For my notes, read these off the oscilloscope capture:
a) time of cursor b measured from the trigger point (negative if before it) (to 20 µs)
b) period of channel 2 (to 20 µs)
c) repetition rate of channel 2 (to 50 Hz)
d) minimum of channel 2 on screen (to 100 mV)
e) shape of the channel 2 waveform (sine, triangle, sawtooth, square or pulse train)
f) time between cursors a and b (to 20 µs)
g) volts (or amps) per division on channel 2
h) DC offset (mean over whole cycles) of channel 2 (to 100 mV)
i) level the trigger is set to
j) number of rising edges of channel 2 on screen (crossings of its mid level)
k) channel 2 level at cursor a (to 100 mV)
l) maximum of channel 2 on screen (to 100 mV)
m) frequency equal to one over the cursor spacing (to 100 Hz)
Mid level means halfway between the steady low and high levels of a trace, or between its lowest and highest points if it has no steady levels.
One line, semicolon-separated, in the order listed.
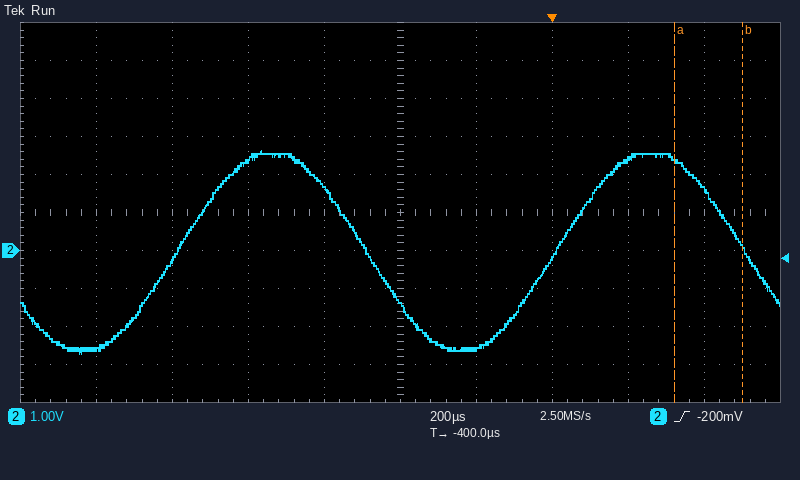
+500 µs; 1.00 ms; 1.00 kHz; -2.7 V; sine; 180 µs; 1 V; 0.0 V; -200 mV; 2; 2.4 V; 2.6 V; 5.6 kHz
